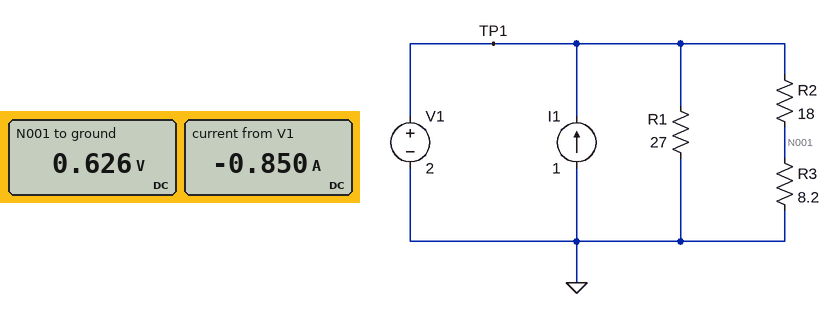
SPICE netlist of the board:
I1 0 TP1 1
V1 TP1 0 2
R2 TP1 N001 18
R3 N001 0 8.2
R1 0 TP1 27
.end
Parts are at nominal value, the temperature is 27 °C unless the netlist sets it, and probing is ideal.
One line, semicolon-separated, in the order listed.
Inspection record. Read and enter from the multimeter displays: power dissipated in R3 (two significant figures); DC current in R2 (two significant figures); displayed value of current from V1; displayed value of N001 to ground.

48 mW; 76 mA; -0.850 A; 0.626 V
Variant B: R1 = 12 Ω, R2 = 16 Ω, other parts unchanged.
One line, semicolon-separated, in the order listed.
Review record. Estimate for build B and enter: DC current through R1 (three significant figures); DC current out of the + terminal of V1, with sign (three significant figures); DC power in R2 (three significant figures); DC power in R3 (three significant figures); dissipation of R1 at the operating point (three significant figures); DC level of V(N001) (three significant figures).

167 mA; -751 mA; 109 mW; 56.0 mW; 333 mW; 678 mV
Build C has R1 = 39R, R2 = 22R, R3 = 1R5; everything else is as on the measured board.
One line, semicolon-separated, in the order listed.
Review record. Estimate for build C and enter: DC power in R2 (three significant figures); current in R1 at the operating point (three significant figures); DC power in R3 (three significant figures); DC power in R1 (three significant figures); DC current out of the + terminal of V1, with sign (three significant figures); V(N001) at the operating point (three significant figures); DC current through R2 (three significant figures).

159 mW; 51.3 mA; 10.9 mW; 103 mW; -864 mA; 128 mV; 85.1 mA
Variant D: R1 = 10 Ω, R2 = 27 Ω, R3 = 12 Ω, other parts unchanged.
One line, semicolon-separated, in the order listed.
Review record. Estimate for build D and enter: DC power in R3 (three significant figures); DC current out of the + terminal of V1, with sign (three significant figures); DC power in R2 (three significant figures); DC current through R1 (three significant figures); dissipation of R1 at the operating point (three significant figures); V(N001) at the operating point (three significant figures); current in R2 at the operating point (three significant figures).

31.6 mW; -749 mA; 71.0 mW; 200 mA; 400 mW; 615 mV; 51.3 mA
